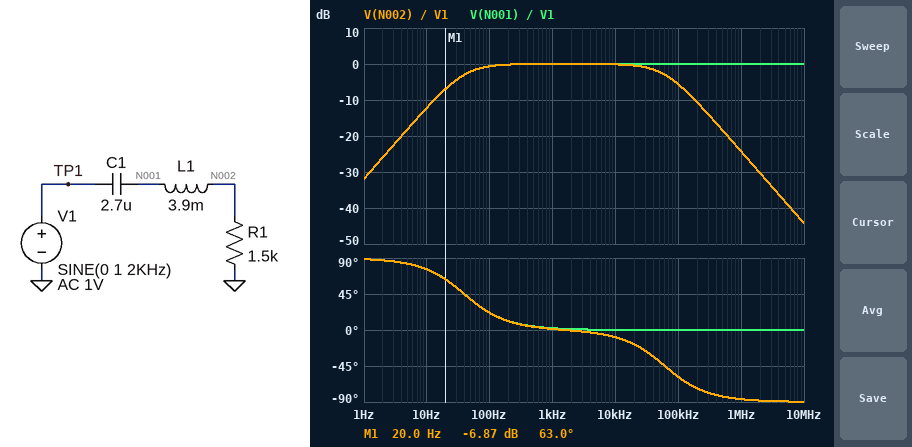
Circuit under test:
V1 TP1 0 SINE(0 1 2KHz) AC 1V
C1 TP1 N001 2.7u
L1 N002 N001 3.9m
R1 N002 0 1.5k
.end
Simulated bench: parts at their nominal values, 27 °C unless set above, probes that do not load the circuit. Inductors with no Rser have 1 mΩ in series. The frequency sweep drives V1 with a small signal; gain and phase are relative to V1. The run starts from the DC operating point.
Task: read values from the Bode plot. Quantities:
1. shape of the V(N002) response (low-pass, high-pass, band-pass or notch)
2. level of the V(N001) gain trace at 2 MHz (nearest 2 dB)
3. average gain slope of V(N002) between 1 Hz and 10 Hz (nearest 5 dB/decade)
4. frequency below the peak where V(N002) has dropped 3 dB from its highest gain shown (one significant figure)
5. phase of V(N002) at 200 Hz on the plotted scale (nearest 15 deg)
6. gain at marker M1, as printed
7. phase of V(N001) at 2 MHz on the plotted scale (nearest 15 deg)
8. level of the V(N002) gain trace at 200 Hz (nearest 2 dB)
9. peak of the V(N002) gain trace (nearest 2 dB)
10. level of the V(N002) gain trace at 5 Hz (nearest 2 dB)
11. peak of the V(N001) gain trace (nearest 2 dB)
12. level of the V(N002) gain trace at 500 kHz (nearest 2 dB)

band-pass
0 dB
20 dB/decade
40 Hz
15 deg
-6.87 dB
0 deg
0 dB
0 dB
-18 dB
0 dB
-18 dB
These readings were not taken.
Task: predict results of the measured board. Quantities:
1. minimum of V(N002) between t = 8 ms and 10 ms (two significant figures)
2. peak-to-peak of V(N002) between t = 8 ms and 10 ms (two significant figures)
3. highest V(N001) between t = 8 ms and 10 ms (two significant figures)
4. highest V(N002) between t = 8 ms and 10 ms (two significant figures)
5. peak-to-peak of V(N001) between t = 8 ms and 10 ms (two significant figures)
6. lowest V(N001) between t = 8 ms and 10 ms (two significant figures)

-1.0 V
2.0 V
1.0 V
1.0 V
2.0 V
-1.0 V
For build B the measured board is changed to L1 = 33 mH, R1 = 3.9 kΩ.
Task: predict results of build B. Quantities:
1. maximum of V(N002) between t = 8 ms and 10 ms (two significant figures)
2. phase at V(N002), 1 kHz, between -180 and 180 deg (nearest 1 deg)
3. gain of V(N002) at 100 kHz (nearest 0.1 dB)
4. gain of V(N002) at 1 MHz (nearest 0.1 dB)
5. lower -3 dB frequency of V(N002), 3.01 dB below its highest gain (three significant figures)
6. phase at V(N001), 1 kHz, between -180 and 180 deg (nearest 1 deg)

990 mV
-2 deg
-14.7 dB
-34.5 dB
15.1 Hz
1 deg
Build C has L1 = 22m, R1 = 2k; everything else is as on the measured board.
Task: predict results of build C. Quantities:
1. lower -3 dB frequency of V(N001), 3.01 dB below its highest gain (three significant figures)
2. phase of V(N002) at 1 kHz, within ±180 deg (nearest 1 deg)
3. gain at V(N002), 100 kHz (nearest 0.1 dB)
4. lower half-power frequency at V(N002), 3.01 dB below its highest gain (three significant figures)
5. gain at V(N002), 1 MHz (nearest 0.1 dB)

29.5 Hz
-2 deg
-16.9 dB
29.4 Hz
-36.8 dB
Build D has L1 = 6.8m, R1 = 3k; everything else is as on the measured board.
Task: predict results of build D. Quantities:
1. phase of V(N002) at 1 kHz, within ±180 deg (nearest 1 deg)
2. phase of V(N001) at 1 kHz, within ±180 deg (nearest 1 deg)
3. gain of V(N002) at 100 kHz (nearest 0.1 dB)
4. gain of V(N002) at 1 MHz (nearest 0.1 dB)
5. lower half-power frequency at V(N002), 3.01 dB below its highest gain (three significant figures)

0 deg
1 deg
-4.8 dB
-23.1 dB
19.6 Hz
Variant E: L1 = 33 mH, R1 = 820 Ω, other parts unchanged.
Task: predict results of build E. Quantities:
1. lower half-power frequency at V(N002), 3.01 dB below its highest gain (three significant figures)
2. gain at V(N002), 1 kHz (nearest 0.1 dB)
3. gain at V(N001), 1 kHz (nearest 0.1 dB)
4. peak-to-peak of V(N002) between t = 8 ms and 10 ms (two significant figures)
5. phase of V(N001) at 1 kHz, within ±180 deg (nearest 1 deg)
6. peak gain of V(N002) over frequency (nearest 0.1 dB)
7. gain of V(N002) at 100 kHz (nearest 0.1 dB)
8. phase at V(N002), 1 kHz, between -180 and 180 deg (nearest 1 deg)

70.6 Hz
-0.1 dB
0.1 dB
1.8 V
4 deg
0 dB
-28.1 dB
-10 deg
